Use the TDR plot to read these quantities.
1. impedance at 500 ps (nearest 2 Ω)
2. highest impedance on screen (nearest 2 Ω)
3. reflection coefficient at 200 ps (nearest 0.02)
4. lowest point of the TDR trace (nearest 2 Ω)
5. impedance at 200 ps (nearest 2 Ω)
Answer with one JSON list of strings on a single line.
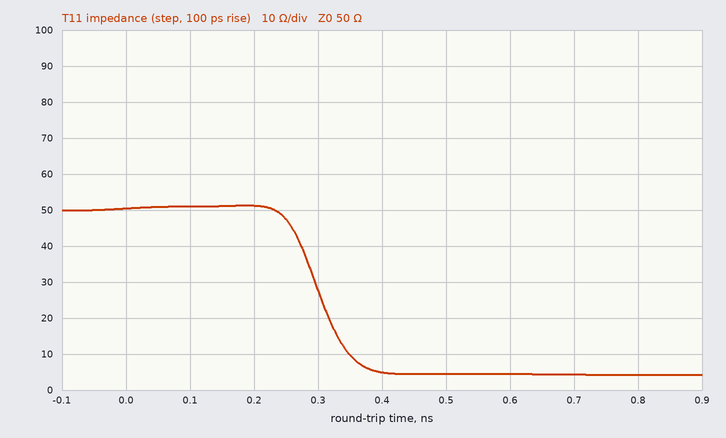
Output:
["4 Ω", "52 Ω", "+0.02", "4 Ω", "52 Ω"]
